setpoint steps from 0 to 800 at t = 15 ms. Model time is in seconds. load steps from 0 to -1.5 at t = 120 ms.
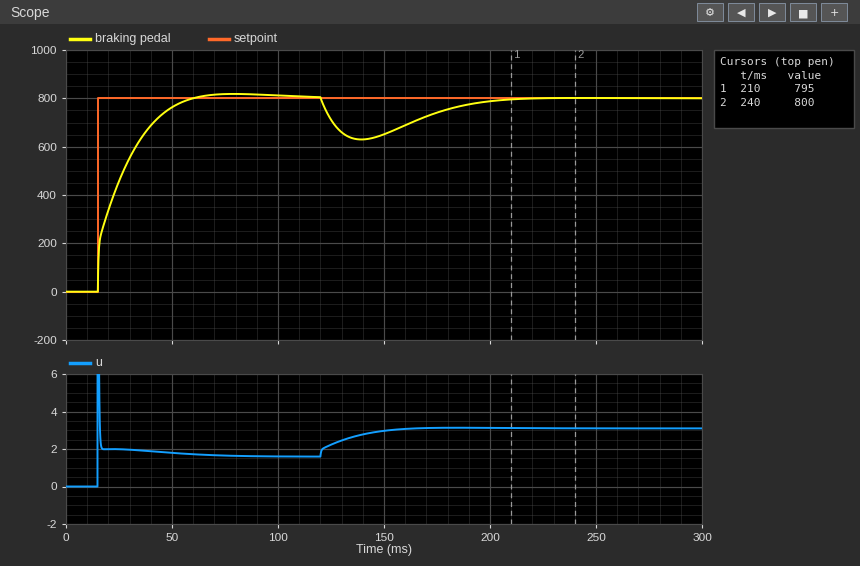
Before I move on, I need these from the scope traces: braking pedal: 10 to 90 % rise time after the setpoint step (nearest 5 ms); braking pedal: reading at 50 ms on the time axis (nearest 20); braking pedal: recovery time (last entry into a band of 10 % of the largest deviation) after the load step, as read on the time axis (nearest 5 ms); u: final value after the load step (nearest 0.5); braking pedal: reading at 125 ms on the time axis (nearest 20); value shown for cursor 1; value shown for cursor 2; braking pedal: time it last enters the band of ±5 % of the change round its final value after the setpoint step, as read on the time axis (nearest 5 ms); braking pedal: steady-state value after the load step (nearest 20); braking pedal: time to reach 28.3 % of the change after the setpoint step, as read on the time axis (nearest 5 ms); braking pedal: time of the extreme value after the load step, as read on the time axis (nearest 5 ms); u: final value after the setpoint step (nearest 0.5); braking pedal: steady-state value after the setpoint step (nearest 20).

30 ms
760
195 ms
3.0
720
795
800
50 ms
800
15 ms
140 ms
1.5
800
